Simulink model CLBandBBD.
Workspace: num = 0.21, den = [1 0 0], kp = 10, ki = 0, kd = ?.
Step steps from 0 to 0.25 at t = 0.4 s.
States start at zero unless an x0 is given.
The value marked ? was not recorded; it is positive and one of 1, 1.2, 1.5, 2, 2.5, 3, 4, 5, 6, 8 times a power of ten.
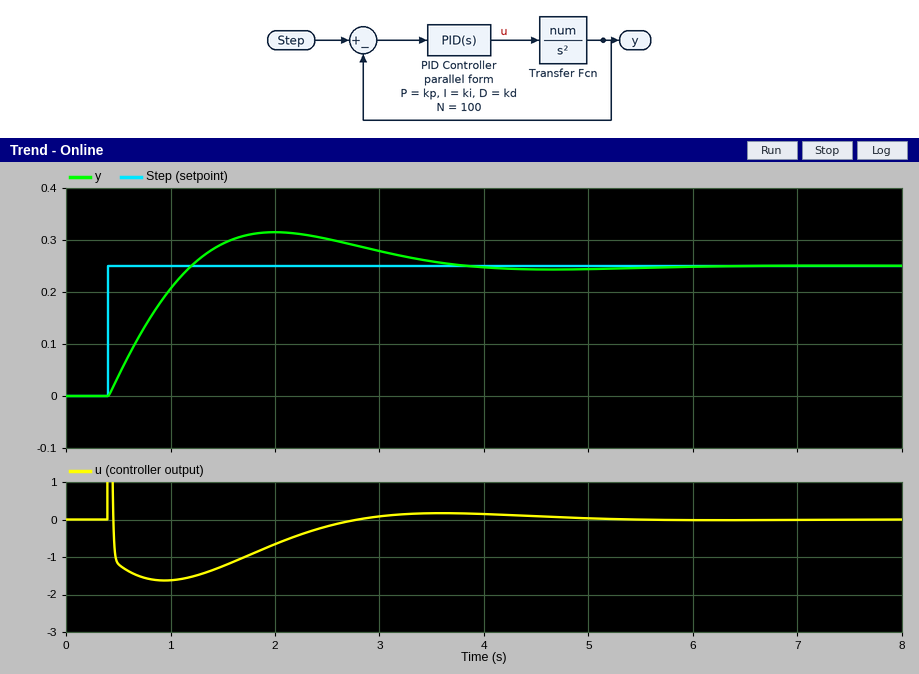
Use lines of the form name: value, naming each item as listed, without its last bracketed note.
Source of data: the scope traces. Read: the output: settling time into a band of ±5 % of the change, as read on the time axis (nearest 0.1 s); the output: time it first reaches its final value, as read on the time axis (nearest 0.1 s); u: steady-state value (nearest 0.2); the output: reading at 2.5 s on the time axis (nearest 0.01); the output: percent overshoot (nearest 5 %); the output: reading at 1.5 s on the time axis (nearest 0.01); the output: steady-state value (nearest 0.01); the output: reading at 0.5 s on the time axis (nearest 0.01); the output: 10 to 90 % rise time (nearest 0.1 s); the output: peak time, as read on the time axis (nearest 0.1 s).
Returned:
the output: settling time into a band of ±5 % of the change, as read on the time axis: 3.4 s
the output: time it first reaches its final value, as read on the time axis: 1.2 s
u: steady-state value: 0.0
the output: reading at 2.5 s on the time axis: 0.30
the output: percent overshoot: 25 %
the output: reading at 1.5 s on the time axis: 0.29
the output: steady-state value: 0.25
the output: reading at 0.5 s on the time axis: 0.04
the output: 10 to 90 % rise time: 0.6 s
the output: peak time, as read on the time axis: 2.0 s
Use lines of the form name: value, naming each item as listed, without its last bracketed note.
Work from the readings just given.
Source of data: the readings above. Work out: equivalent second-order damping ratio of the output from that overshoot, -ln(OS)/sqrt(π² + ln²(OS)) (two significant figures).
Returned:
equivalent second-order damping ratio of the output from that overshoot, -ln(OS)/sqrt(π² + ln²(OS)): 0.40
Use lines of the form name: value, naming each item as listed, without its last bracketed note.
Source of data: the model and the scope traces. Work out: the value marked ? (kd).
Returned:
the value marked ?: 8
